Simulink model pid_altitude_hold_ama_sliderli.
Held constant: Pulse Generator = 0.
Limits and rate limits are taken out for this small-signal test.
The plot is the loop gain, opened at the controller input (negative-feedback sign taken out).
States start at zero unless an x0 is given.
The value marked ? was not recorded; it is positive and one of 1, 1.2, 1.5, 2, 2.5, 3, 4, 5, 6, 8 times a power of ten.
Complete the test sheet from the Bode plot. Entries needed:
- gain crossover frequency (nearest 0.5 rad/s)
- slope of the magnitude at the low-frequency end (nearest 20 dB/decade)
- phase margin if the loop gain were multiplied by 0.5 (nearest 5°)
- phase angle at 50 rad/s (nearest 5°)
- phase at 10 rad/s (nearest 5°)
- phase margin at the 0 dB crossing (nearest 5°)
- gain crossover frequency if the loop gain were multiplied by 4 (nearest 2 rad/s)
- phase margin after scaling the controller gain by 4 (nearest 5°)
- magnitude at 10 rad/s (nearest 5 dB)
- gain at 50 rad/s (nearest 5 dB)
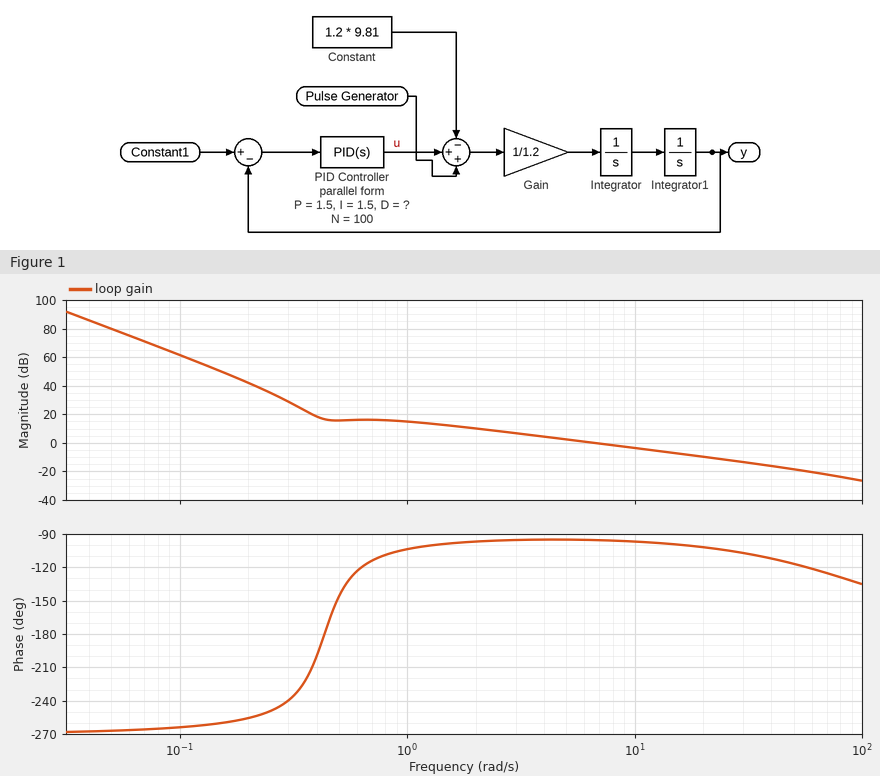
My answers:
6.5 rad/s
-60 dB/decade
85°
-115°
-95°
85°
26 rad/s
75°
-5 dB
-20 dB
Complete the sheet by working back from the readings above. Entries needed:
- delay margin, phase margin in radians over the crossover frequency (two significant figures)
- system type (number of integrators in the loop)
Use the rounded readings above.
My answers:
0.23 s
3
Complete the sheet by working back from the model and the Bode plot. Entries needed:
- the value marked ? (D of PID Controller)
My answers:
8
